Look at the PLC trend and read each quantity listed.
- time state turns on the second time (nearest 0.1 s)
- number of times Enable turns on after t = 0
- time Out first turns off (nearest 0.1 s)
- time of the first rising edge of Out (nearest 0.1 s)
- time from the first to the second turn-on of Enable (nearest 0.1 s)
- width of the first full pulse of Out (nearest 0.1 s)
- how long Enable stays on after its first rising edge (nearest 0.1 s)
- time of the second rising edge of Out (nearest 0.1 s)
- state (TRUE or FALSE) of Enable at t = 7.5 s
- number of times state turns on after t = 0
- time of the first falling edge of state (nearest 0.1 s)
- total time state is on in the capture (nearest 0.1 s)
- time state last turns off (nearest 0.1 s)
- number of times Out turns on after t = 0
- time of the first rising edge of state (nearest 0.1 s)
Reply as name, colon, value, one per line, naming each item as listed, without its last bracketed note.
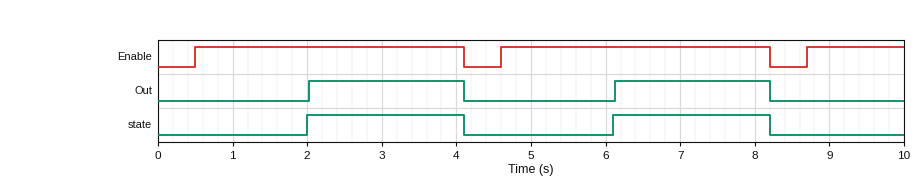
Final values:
time state turns on the second time: 6.1 s
number of times Enable turns on after t = 0: 3
time Out first turns off: 4.1 s
time of the first rising edge of Out: 2.0 s
time from the first to the second turn-on of Enable: 4.1 s
width of the first full pulse of Out: 2.1 s
how long Enable stays on after its first rising edge: 3.6 s
time of the second rising edge of Out: 6.1 s
state (TRUE or FALSE) of Enable at t = 7.5 s: TRUE
number of times state turns on after t = 0: 2
time of the first falling edge of state: 4.1 s
total time state is on in the capture: 4.2 s
time state last turns off: 8.2 s
number of times Out turns on after t = 0: 2
time of the first rising edge of state: 2.0 s
